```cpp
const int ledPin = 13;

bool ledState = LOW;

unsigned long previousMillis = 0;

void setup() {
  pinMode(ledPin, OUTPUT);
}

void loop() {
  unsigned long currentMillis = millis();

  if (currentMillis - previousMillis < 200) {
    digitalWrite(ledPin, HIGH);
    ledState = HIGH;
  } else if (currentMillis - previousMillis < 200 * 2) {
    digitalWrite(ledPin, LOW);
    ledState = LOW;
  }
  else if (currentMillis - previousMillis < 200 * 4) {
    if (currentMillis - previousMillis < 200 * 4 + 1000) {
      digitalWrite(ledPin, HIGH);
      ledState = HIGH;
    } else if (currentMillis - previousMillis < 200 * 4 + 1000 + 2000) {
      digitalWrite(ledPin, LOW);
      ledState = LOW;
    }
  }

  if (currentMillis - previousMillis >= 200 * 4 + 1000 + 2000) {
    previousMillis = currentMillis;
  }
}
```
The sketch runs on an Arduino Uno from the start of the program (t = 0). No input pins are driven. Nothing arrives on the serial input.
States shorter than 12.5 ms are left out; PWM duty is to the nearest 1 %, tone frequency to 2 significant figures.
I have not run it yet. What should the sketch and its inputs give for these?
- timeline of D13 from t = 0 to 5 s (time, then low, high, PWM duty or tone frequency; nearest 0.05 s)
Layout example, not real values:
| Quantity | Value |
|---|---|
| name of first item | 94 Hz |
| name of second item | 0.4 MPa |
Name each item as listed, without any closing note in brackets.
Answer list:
| Quantity | Value |
|---|---|
| timeline of D13 from t = 0 to 5 s | 0 s high; 0.2 s low; 0.4 s high; 4 s low; 4.2 s high |
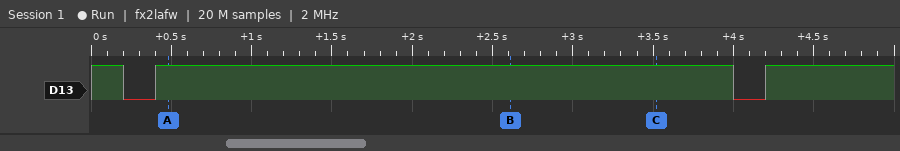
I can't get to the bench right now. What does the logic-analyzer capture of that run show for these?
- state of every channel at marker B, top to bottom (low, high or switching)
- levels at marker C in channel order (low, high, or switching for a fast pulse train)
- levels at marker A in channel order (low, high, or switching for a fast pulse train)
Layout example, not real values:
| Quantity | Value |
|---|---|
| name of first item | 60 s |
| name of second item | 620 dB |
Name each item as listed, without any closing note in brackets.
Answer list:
| Quantity | Value |
|---|---|
| state of every channel at marker B, top to bottom | D13 high |
| levels at marker C in channel order | D13 high |
| levels at marker A in channel order | D13 high |
